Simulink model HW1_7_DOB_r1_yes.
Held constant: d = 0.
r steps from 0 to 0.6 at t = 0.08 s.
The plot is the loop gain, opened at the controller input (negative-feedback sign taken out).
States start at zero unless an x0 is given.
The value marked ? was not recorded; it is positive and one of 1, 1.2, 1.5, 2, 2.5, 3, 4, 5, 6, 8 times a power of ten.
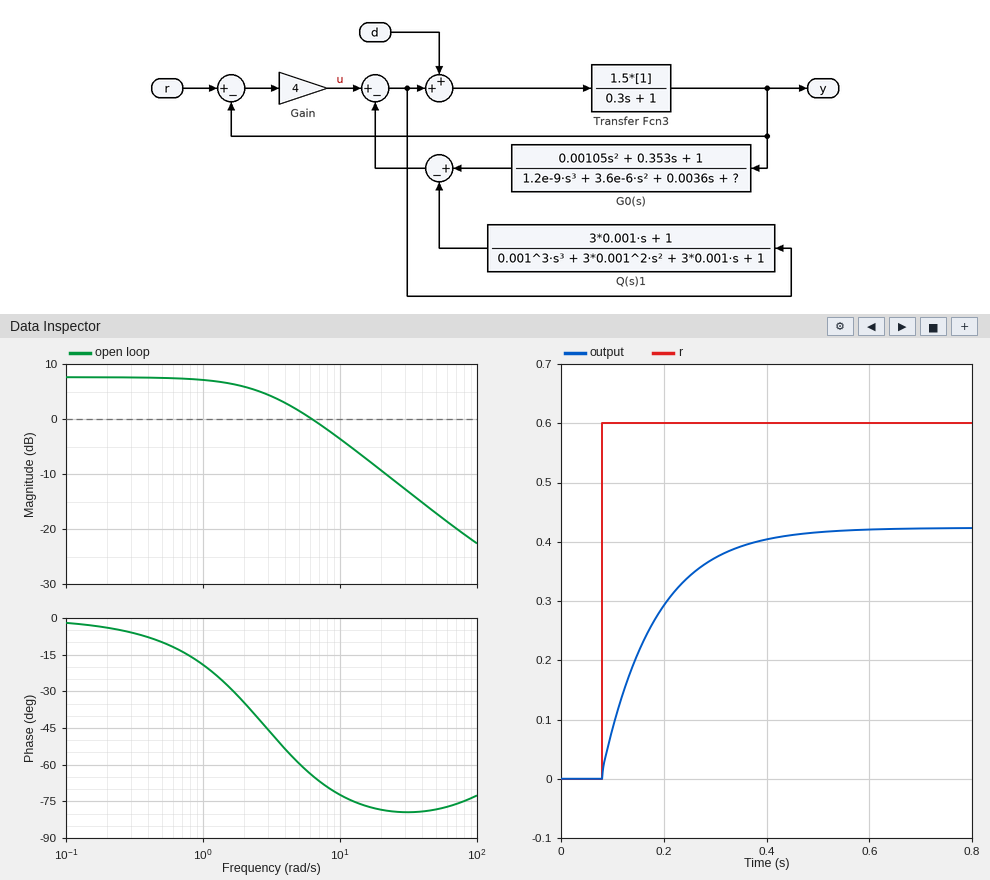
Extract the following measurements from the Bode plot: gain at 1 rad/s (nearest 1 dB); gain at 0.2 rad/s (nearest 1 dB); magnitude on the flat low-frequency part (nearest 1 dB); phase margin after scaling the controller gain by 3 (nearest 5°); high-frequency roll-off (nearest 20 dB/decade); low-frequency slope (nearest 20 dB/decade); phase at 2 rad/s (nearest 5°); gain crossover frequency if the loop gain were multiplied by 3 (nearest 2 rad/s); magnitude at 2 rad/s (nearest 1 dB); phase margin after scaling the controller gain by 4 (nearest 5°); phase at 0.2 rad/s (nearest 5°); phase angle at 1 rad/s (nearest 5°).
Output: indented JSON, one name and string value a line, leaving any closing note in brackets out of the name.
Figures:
{
  "gain at 1 rad/s": "7 dB",
  "gain at 0.2 rad/s": "8 dB",
  "magnitude on the flat low-frequency part": "8 dB",
  "phase margin after scaling the controller gain by 3": "100°",
  "high-frequency roll-off": "-20 dB/decade",
  "low-frequency slope": "0 dB/decade",
  "phase at 2 rad/s": "-35°",
  "gain crossover frequency if the loop gain were multiplied by 3": "20 rad/s",
  "magnitude at 2 rad/s": "6 dB",
  "phase margin after scaling the controller gain by 4": "100°",
  "phase at 0.2 rad/s": "-5°",
  "phase angle at 1 rad/s": "-20°"
}
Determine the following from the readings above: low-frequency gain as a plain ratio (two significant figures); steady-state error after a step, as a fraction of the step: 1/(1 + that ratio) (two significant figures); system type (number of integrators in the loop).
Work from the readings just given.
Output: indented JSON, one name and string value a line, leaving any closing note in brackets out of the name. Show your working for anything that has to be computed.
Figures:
{
  "low-frequency gain as a plain ratio": "10^(8 / 20) = 2.5",
  "steady-state error after a step, as a fraction of the step: 1/(1 + that ratio)": "1 / (1 + 2.5) = 0.29",
  "system type": "0"
}
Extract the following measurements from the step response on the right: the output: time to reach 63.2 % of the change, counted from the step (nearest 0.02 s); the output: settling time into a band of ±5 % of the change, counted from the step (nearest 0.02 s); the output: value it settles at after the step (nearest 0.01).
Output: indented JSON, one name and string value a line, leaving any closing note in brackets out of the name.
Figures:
{
  "the output: time to reach 63.2 % of the change, counted from the step": "0.10 s",
  "the output: settling time into a band of ±5 % of the change, counted from the step": "0.32 s",
  "the output: value it settles at after the step": "0.42"
}
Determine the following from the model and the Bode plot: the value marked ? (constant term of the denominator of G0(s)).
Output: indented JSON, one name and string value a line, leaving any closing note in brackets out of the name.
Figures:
{
  "the value marked ? (constant term of the denominator of G0(s))": "0.6"
}
